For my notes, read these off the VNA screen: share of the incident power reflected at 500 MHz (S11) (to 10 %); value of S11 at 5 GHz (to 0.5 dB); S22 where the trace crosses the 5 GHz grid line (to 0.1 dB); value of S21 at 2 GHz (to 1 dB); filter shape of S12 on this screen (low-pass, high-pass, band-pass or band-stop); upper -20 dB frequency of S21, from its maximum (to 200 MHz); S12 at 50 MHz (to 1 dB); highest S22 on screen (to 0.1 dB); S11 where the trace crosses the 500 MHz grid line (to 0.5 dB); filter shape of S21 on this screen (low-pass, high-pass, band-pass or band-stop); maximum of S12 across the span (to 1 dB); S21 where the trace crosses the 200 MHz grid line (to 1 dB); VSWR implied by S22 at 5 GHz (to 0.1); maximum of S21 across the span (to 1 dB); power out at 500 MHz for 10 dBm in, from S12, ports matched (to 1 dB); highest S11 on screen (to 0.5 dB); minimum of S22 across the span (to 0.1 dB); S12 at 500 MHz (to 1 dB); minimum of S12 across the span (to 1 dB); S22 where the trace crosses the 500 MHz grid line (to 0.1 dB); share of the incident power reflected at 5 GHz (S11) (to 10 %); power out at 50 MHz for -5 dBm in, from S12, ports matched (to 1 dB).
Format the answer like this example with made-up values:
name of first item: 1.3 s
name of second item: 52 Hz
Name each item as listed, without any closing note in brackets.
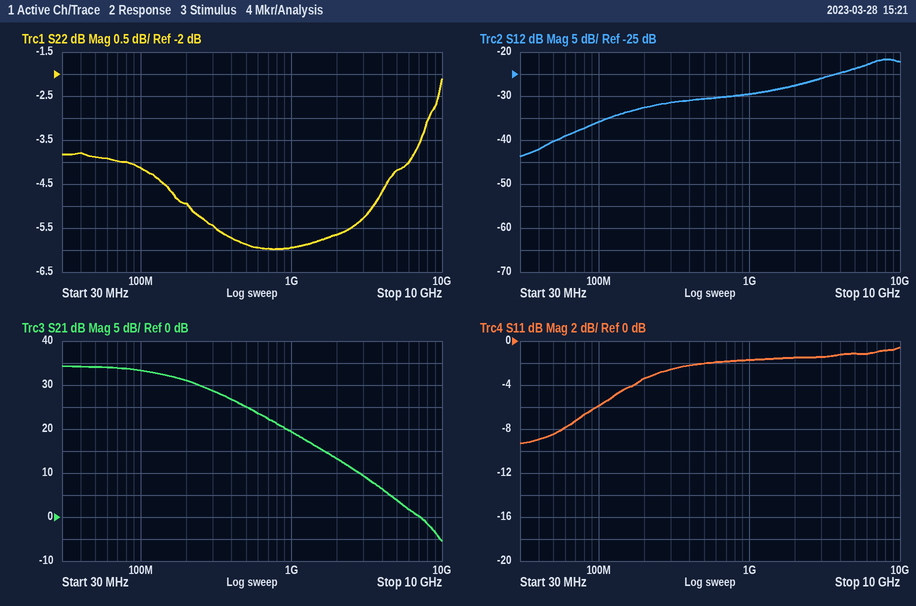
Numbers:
share of the incident power reflected at 500 MHz (S11): 60 %
value of S11 at 5 GHz: -1.0 dB
S22 where the trace crosses the 5 GHz grid line: -4.2 dB
value of S21 at 2 GHz: 13 dB
filter shape of S12 on this screen: high-pass
upper -20 dB frequency of S21, from its maximum: 1.8 GHz
S12 at 50 MHz: -40 dB
highest S22 on screen: -2.1 dB
S11 where the trace crosses the 500 MHz grid line: -2.0 dB
filter shape of S21 on this screen: low-pass
maximum of S12 across the span: -22 dB
S21 where the trace crosses the 200 MHz grid line: 31 dB
VSWR implied by S22 at 5 GHz: 4.2
maximum of S21 across the span: 34 dB
power out at 500 MHz for 10 dBm in, from S12, ports matched: -21 dBm
highest S11 on screen: -0.5 dB
minimum of S22 across the span: -6.0 dB
S12 at 500 MHz: -31 dB
minimum of S12 across the span: -44 dB
S22 where the trace crosses the 500 MHz grid line: -5.9 dB
share of the incident power reflected at 5 GHz (S11): 80 %
power out at 50 MHz for -5 dBm in, from S12, ports matched: -45 dBm
